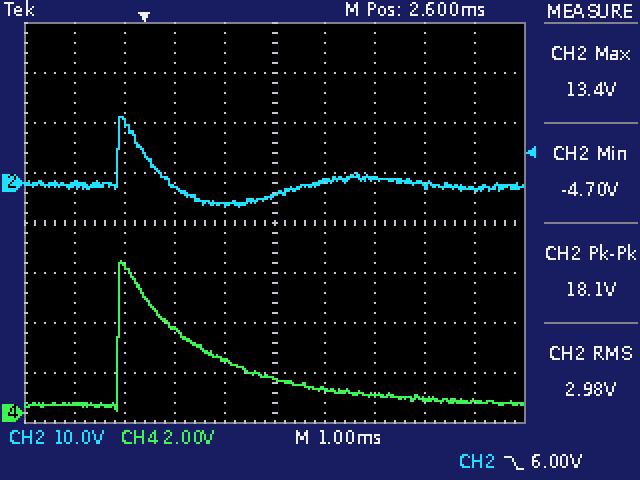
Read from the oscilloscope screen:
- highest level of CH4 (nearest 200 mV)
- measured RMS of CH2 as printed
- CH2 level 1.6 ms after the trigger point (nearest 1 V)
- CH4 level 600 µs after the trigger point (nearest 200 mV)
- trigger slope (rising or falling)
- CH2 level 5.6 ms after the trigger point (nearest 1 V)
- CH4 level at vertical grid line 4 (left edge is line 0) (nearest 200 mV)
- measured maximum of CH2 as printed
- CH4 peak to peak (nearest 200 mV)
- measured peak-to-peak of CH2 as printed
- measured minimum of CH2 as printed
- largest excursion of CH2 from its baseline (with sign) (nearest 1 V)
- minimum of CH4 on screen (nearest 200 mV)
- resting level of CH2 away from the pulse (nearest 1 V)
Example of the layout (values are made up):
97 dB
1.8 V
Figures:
6.0 V
2.98 V
-4 V
3.4 V
falling
0 V
2.2 V
13.4 V
6.0 V
18.1 V
-4.70 V
+14 V
0.0 V
0 V
